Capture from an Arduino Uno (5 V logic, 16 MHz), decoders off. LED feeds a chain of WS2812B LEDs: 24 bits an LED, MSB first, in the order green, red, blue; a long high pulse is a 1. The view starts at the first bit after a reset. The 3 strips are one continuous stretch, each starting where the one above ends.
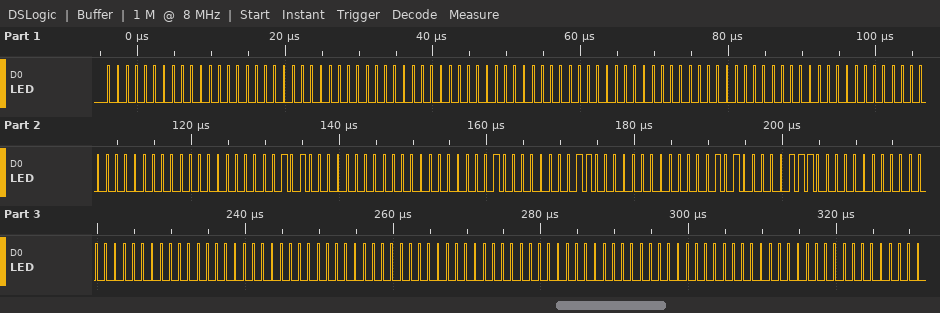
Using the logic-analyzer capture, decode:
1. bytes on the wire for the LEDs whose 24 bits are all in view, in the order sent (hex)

00 00 00 00 00 00 00 00 00 00 00 00 00 05 00 00 08 06 00 0A 0E 00 00 00 00 00 00 00 00 00 00 00 00
